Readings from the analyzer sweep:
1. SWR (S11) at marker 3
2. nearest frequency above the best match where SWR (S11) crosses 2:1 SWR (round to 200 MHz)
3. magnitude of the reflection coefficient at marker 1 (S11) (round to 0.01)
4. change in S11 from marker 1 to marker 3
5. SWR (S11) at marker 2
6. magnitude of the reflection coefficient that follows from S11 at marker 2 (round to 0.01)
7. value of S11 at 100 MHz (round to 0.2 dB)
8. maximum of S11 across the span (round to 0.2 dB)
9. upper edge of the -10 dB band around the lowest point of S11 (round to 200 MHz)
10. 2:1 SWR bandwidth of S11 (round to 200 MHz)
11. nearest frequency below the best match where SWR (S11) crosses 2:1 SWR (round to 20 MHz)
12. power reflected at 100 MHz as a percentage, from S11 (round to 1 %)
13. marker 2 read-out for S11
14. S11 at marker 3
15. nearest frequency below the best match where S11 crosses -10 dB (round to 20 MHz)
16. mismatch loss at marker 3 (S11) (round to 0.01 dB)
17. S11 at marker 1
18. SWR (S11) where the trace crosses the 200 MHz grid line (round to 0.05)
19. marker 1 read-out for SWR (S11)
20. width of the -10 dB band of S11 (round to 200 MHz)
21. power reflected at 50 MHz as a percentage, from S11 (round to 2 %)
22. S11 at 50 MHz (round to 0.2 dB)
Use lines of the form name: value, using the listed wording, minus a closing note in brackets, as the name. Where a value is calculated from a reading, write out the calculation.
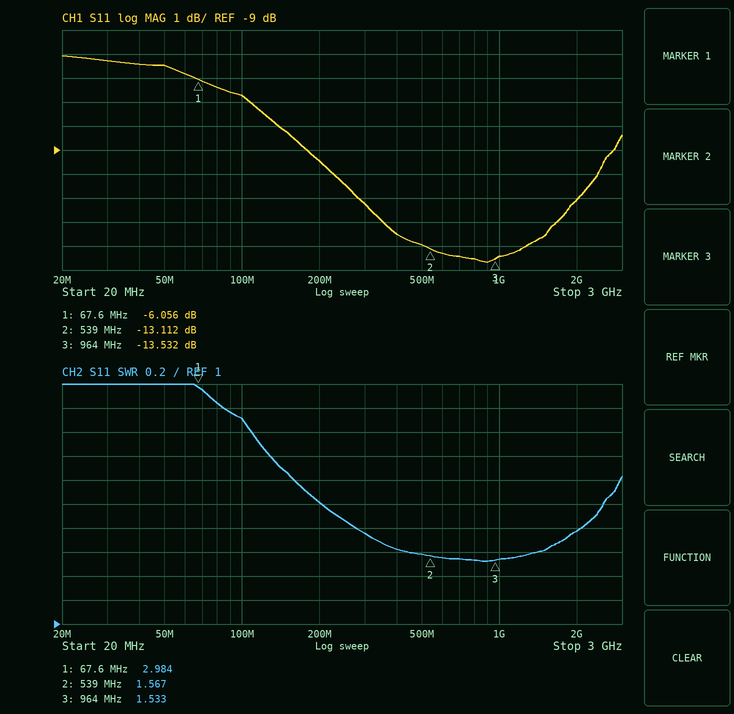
SWR (S11) at marker 3: 1.533
nearest frequency above the best match where SWR (S11) crosses 2:1 SWR: 2.6 GHz
magnitude of the reflection coefficient at marker 1 (S11): 10^(-6.056/20) ≈ 0.50
change in S11 from marker 1 to marker 3: -13.532 − (-6.056) = -7.476 dB
SWR (S11) at marker 2: 1.567
magnitude of the reflection coefficient that follows from S11 at marker 2: 10^(-13.112/20) ≈ 0.22
value of S11 at 100 MHz: -6.8 dB
maximum of S11 across the span: -5.0 dB
upper edge of the -10 dB band around the lowest point of S11: 2.4 GHz
2:1 SWR bandwidth of S11: 2.6 GHz − 200 MHz = 2.40 GHz
nearest frequency below the best match where SWR (S11) crosses 2:1 SWR: 200 MHz
power reflected at 100 MHz as a percentage, from S11: 10^(-6.8/10) ≈ 21 %
marker 2 read-out for S11: -13.112 dB
S11 at marker 3: -13.532 dB
nearest frequency below the best match where S11 crosses -10 dB: 220 MHz
mismatch loss at marker 3 (S11): −10 log10(1 − 10^(-13.532/10)) ≈ 0.20 dB
S11 at marker 1: -6.056 dB
SWR (S11) where the trace crosses the 200 MHz grid line: 2.00
marker 1 read-out for SWR: 2.984
width of the -10 dB band of S11: 2.4 GHz − 220 MHz = 2.18 GHz
power reflected at 50 MHz as a percentage, from S11: 10^(-5.4/10) ≈ 28.8 %, so 28 % to the nearest 2 %
S11 at 50 MHz: -5.4 dB
